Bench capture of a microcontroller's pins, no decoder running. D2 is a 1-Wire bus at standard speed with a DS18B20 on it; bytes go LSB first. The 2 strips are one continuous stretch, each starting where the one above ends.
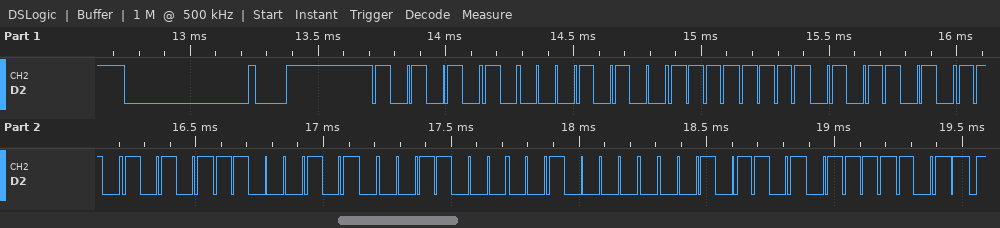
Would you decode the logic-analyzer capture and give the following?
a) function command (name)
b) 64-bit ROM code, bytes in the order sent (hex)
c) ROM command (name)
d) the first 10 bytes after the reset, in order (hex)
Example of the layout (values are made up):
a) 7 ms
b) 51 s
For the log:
a) Read Scratchpad
b) 28 FF 5A AB A3 18 04 B4
c) Match ROM
d) 55 28 FF 5A AB A3 18 04 B4 BE
